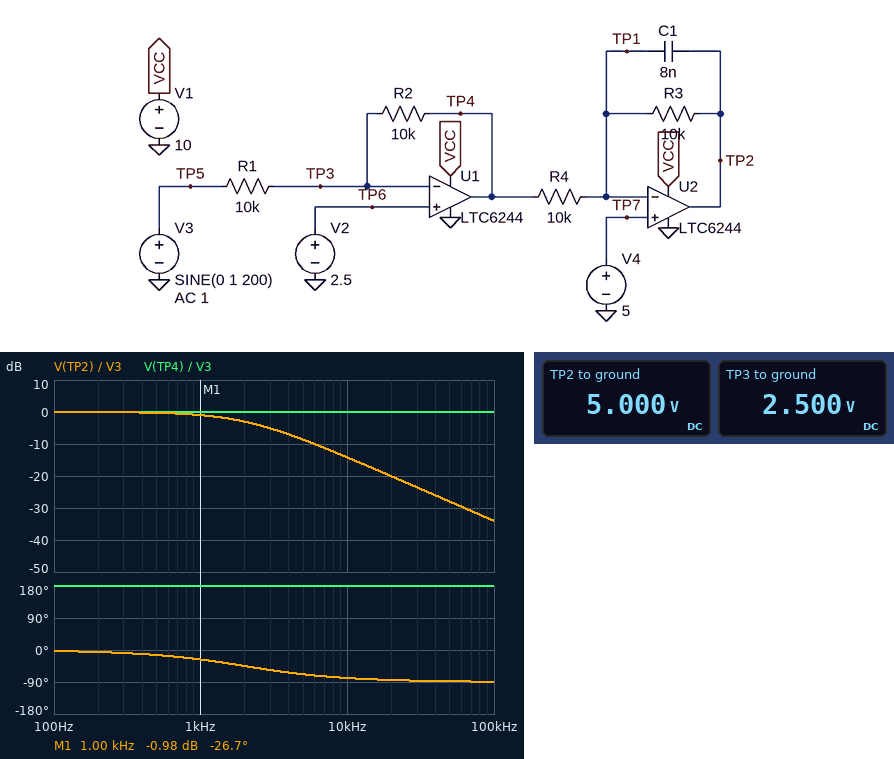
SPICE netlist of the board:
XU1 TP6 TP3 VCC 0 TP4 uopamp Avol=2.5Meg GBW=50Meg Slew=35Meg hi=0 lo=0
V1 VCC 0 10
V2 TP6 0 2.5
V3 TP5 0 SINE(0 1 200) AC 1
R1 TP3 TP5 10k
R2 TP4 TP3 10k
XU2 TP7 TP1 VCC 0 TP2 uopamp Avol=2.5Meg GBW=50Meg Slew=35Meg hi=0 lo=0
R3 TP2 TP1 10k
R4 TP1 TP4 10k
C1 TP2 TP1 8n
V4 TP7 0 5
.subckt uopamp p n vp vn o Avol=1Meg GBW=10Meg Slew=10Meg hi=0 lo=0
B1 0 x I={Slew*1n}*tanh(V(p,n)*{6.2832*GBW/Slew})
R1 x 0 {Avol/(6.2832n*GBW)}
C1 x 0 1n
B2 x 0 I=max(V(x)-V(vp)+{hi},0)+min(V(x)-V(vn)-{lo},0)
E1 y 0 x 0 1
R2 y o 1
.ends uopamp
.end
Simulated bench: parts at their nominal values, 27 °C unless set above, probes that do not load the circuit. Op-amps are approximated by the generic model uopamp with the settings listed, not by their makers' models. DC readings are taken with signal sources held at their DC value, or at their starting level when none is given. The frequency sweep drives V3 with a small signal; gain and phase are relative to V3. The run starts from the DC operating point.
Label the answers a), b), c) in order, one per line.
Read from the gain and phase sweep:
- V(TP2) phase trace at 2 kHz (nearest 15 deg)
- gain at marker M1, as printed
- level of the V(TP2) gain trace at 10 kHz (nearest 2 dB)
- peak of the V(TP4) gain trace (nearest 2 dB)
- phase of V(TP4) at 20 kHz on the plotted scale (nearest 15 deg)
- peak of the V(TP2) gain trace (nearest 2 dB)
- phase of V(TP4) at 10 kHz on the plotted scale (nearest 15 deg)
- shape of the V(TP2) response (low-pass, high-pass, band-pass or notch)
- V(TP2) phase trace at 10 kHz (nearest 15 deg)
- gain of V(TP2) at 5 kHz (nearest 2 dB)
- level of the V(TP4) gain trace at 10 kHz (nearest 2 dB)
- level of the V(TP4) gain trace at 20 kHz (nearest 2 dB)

a) -45 deg
b) -0.98 dB
c) -14 dB
d) 0 dB
e) 180 deg
f) 0 dB
g) 180 deg
h) low-pass
i) -75 deg
j) -8 dB
k) 0 dB
l) 0 dB
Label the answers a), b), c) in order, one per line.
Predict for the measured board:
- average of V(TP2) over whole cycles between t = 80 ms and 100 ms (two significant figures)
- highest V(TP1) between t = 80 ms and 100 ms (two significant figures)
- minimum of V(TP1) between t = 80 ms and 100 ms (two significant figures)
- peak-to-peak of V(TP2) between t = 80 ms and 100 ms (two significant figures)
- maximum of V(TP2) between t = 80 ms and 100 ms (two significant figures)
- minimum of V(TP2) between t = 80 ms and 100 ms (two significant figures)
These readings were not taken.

a) 5.0 V
b) 5.0 V
c) 5.0 V
d) 2.0 V
e) 6.0 V
f) 4.0 V
